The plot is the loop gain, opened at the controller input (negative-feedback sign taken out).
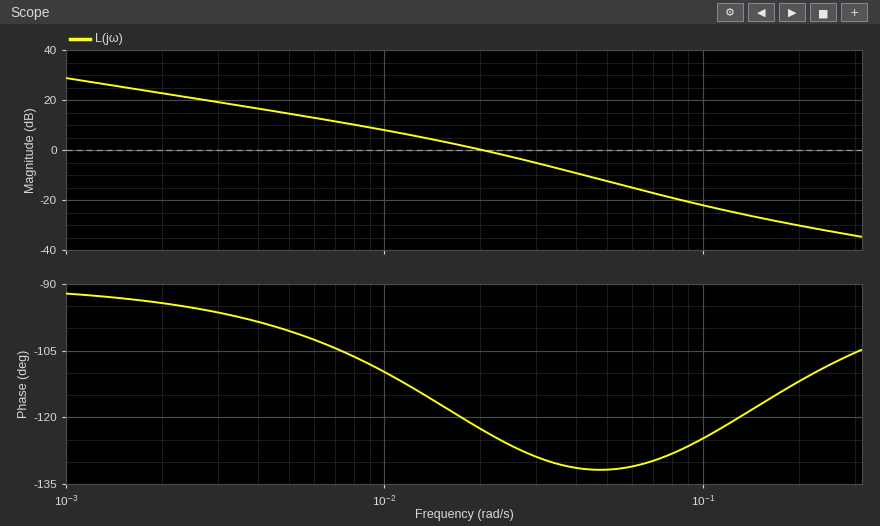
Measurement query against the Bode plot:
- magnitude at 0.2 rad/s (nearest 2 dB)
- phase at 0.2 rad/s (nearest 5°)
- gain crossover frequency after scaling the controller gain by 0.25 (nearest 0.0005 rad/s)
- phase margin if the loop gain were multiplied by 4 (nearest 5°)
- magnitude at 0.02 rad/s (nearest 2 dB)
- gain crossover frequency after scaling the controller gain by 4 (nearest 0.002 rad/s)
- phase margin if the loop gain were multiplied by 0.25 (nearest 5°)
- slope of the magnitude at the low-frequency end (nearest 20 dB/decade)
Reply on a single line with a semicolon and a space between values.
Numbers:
-30 dB; -110°; 0.0065 rad/s; 50°; 0 dB; 0.048 rad/s; 75°; -20 dB/decade
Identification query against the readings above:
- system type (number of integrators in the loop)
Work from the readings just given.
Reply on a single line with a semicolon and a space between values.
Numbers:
1
